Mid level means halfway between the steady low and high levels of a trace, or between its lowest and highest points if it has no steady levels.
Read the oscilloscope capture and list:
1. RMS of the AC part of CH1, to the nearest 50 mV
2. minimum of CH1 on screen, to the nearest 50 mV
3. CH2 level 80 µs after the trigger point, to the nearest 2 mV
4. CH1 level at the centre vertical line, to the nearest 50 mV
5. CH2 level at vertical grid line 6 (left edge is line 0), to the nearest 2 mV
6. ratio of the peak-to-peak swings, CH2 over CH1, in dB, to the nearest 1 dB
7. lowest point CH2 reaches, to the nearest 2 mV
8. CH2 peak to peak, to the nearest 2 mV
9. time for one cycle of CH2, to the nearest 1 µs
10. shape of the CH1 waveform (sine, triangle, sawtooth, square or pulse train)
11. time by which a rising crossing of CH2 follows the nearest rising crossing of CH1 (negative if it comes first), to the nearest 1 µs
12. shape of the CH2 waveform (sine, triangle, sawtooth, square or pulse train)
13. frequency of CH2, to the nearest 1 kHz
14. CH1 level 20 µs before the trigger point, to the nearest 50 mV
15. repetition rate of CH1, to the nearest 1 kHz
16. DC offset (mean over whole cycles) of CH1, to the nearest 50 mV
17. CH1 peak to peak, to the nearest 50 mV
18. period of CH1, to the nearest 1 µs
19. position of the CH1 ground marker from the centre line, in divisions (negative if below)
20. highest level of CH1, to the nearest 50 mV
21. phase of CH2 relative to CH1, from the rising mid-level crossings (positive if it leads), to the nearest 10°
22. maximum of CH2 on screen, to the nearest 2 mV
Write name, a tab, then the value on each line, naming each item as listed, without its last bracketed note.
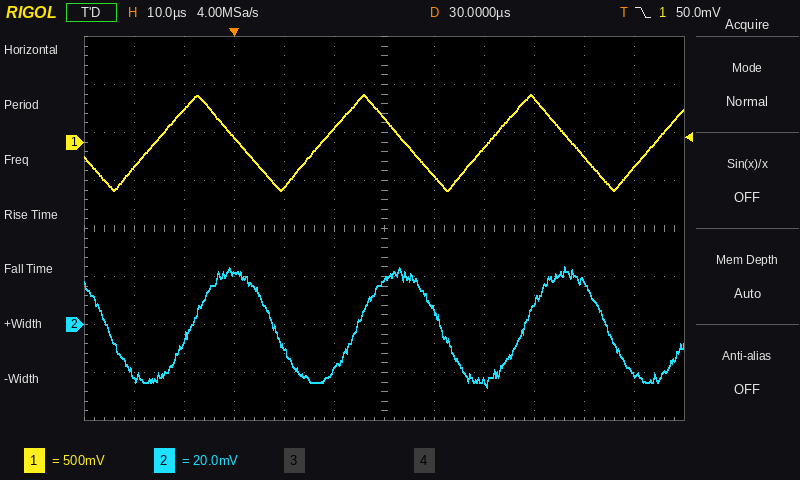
RMS of the AC part of CH1, to the nearest 50 mV	300 mV
minimum of CH1 on screen, to the nearest 50 mV	-500 mV
CH2 level 80 µs after the trigger point, to the nearest 2 mV	-20 mV
CH1 level at the centre vertical line, to the nearest 50 mV	250 mV
CH2 level at vertical grid line 6 (left edge is line 0), to the nearest 2 mV	18 mV
ratio of the peak-to-peak swings, CH2 over CH1, in dB, to the nearest 1 dB	-26 dB
lowest point CH2 reaches, to the nearest 2 mV	-26 mV
CH2 peak to peak, to the nearest 2 mV	50 mV
time for one cycle of CH2, to the nearest 1 µs	33 µs
shape of the CH1 waveform	triangle
time by which a rising crossing of CH2 follows the nearest rising crossing of CH1 (negative if it comes first), to the nearest 1 µs	+7 µs
shape of the CH2 waveform	sine
frequency of CH2, to the nearest 1 kHz	30 kHz
CH1 level 20 µs before the trigger point, to the nearest 50 mV	-250 mV
repetition rate of CH1, to the nearest 1 kHz	30 kHz
DC offset (mean over whole cycles) of CH1, to the nearest 50 mV	0 mV
CH1 peak to peak, to the nearest 50 mV	1.00 V
period of CH1, to the nearest 1 µs	33 µs
position of the CH1 ground marker from the centre line, in divisions	+1.8 div
highest level of CH1, to the nearest 50 mV	500 mV
phase of CH2 relative to CH1, from the rising mid-level crossings (positive if it leads), to the nearest 10°	-80°
maximum of CH2 on screen, to the nearest 2 mV	24 mV
